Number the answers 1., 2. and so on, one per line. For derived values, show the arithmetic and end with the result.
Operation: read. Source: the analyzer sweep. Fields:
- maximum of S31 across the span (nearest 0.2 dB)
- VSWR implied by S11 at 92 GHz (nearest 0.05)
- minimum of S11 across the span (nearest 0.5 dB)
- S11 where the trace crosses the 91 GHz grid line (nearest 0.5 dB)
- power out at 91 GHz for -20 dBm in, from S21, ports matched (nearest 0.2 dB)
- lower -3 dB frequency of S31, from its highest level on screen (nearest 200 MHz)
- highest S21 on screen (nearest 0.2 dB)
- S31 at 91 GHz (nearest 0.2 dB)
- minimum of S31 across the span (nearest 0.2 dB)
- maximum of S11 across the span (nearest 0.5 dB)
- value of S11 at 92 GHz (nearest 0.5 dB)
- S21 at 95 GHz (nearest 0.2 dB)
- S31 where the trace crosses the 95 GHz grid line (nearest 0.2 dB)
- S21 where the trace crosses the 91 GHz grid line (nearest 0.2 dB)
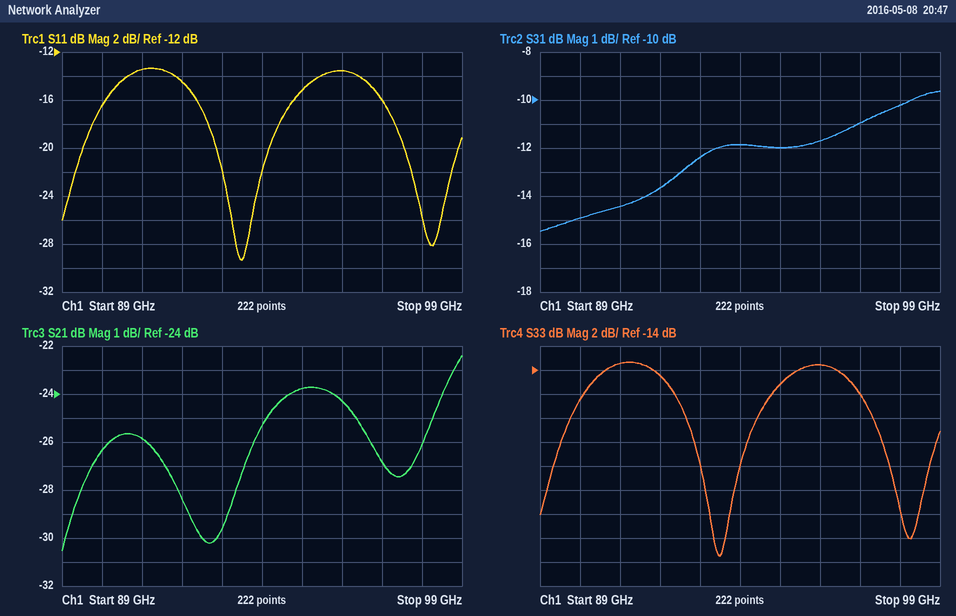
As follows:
1. -9.6 dB
2. |Γ| = 10^(-14.5/20) = 0.1884; VSWR = (1 + 0.1884)/(1 − 0.1884) ≈ 1.46, so 1.45 to the nearest 0.05
3. -29.5 dB
4. -13.5 dB
5. -20 dBm + (-25.8 dB) = -45.8 dBm
6. 92.8 GHz
7. -22.4 dB
8. -14.4 dB
9. -15.4 dB
10. -13.5 dB
11. -14.5 dB
12. -23.8 dB
13. -12.0 dB
14. -25.8 dB
